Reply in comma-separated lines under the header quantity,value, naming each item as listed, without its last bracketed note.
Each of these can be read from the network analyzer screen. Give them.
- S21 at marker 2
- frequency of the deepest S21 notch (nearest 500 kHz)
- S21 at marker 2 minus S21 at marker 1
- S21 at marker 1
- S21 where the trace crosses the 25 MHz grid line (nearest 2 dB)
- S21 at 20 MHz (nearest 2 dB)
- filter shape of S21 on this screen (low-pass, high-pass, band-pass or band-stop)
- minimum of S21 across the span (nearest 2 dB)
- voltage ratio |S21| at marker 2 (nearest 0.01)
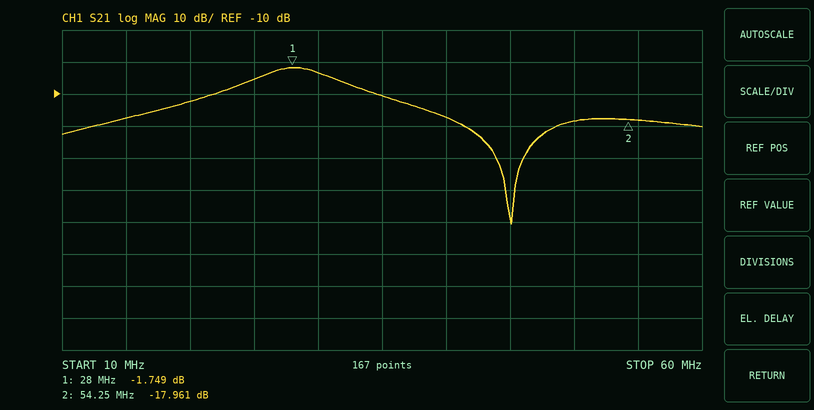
quantity,value
S21 at marker 2,-17.961 dB
frequency of the deepest S21 notch,45.0 MHz
S21 at marker 2 minus S21 at marker 1,-16.212 dB
S21 at marker 1,-1.749 dB
S21 where the trace crosses the 25 MHz grid line,-6 dB
S21 at 20 MHz,-12 dB
filter shape of S21 on this screen,band-pass
minimum of S21 across the span,-50 dB
voltage ratio |S21| at marker 2,0.13
